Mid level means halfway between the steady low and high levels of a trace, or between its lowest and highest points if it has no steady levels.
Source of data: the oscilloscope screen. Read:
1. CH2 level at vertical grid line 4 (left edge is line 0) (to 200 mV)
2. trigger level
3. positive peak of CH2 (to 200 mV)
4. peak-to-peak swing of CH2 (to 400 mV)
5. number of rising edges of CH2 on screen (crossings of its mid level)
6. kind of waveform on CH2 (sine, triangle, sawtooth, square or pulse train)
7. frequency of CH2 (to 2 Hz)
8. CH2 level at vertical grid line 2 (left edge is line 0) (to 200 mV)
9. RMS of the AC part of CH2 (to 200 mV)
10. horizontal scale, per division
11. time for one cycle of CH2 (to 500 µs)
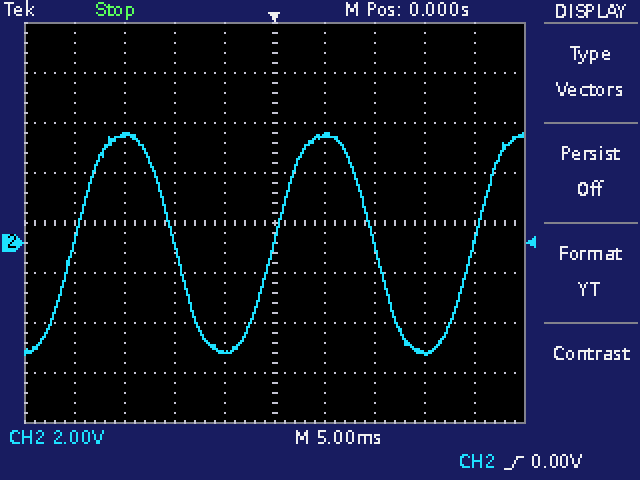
-4.4 V
0.00 V
4.4 V
8.8 V
3
sine
50 Hz
4.4 V
3.2 V
5 ms
20.0 ms
